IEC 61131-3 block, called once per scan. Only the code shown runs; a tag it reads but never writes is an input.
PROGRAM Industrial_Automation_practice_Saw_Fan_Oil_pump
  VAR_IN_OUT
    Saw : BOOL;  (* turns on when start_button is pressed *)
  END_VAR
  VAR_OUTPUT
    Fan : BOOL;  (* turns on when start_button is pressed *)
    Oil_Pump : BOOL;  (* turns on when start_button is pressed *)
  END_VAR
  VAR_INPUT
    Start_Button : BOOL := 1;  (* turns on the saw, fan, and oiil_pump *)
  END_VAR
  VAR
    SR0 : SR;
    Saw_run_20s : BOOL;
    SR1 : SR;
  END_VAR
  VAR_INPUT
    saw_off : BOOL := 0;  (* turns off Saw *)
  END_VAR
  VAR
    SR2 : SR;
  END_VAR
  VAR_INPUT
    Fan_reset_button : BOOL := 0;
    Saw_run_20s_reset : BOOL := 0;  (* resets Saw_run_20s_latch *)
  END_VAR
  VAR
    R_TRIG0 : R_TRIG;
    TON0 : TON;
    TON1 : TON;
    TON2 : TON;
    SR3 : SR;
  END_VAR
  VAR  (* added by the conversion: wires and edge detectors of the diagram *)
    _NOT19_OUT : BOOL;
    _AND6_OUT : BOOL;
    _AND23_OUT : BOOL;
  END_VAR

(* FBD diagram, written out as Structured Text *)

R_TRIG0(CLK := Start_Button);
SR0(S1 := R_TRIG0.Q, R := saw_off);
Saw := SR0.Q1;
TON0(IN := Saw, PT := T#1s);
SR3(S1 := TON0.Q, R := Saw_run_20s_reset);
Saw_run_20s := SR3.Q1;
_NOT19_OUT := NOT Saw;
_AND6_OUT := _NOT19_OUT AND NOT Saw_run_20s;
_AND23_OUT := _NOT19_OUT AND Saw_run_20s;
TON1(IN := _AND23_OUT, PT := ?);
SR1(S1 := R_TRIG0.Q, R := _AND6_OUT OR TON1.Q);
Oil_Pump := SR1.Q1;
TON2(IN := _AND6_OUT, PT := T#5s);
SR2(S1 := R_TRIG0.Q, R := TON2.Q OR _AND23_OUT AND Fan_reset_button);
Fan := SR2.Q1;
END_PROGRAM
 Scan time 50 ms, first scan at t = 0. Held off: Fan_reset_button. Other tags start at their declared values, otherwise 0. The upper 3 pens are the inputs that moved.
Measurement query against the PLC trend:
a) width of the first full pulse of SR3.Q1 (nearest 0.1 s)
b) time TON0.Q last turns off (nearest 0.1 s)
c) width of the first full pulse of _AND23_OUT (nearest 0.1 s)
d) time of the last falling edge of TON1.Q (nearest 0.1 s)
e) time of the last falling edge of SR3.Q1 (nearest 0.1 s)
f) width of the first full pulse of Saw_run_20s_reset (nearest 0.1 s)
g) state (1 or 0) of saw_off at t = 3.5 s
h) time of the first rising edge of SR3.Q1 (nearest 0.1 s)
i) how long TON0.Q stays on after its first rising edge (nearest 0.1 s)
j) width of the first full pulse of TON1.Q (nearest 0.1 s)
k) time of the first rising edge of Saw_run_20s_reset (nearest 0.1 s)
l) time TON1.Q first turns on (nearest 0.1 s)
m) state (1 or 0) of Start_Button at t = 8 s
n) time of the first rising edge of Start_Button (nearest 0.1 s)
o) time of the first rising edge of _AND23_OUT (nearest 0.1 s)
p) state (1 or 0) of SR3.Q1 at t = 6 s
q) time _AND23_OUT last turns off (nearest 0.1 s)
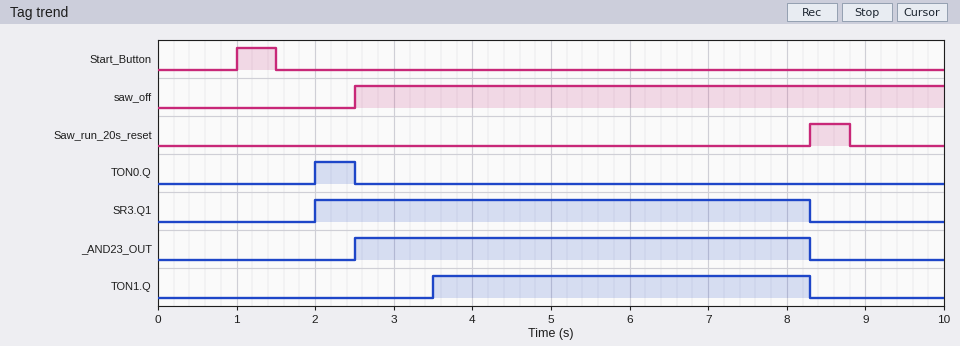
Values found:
6.3 s
2.5 s
5.8 s
8.3 s
8.3 s
0.5 s
1
2.0 s
0.5 s
4.8 s
8.3 s
3.5 s
0
1.0 s
2.5 s
1
8.3 s
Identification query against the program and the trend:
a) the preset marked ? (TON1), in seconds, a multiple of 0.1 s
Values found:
1.0 s
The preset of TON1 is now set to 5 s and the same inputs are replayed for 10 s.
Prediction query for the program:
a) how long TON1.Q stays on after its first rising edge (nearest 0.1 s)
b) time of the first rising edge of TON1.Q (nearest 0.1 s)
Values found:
0.8 s
7.5 s
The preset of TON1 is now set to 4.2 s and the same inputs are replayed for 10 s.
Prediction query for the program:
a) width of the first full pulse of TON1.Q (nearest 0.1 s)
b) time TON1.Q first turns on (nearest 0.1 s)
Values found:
1.6 s
6.7 s
